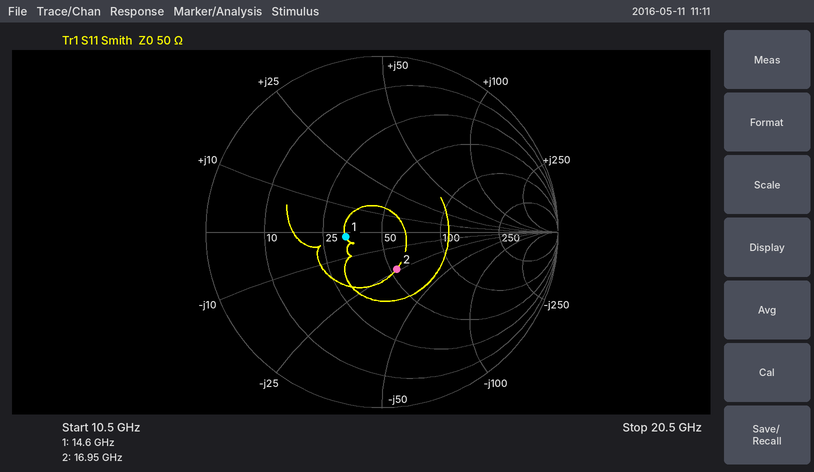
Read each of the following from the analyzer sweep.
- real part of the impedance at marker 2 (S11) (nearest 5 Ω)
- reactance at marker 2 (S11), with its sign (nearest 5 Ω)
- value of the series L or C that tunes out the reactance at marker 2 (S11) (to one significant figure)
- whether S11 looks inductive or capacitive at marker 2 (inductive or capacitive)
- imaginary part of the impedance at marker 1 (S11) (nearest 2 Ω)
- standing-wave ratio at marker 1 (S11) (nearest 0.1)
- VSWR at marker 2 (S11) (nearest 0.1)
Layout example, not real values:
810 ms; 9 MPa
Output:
55 Ω; -25 Ω; 200 pH; capacitive; -2 Ω; 1.5; 1.6
